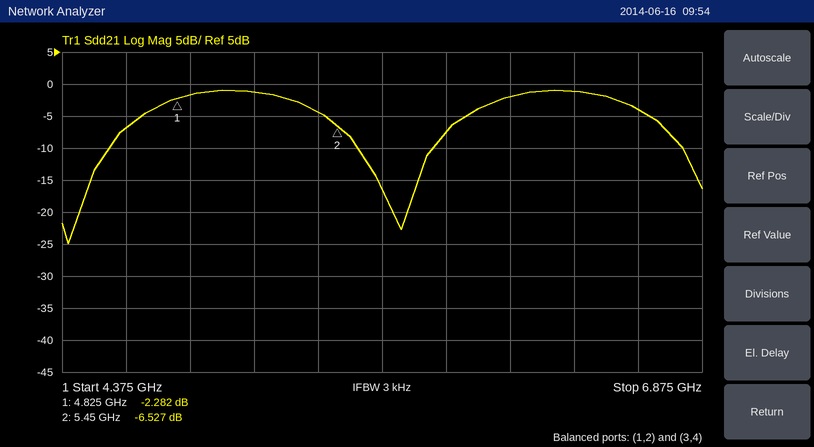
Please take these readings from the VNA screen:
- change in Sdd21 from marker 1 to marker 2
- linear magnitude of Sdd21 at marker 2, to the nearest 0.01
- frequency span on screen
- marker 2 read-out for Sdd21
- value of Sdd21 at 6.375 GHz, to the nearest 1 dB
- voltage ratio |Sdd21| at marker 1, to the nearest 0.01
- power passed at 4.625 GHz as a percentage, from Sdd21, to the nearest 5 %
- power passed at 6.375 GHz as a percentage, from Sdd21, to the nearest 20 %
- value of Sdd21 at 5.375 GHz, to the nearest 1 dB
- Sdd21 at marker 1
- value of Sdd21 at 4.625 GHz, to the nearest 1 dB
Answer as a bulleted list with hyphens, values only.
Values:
- -4.245 dB
- 0.47
- 2.5 GHz
- -6.527 dB
- -1 dB
- 0.77
- 20 %
- 80 %
- -4 dB
- -2.282 dB
- -7 dB
